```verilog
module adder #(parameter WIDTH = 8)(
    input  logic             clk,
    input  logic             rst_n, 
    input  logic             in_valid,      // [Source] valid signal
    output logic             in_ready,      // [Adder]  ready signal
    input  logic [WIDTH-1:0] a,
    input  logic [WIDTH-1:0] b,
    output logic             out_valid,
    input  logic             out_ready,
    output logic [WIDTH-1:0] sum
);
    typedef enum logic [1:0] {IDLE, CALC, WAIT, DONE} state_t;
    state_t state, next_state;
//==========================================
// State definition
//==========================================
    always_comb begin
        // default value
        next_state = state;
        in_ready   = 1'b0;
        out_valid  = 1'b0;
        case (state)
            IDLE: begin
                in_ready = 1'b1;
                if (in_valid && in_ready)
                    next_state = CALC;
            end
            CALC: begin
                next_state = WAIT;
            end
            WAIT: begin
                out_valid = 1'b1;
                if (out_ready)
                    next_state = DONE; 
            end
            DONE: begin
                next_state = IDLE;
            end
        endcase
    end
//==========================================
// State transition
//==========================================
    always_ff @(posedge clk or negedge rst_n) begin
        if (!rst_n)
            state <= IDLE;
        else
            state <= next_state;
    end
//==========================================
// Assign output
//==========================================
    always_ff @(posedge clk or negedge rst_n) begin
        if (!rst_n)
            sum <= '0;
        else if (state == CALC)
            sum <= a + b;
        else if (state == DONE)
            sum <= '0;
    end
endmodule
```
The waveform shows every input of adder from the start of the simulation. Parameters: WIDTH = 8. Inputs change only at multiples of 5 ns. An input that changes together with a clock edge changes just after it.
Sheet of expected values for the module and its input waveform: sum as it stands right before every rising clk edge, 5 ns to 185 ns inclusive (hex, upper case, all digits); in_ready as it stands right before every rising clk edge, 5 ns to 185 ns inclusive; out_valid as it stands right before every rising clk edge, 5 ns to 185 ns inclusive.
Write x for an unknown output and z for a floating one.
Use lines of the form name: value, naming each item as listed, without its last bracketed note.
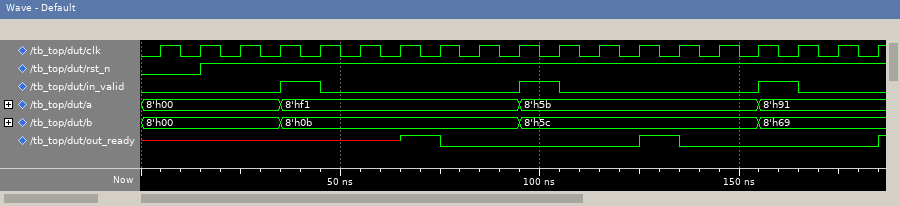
sum as it stands right before every rising clk edge, 5 ns to 185 ns inclusive: 00, 00, 00, 00, 00, 00, FC, FC, FC, 00, 00, 00, B7, B7, B7, 00, 00, 00, FA
in_ready as it stands right before every rising clk edge, 5 ns to 185 ns inclusive: 1 1 1 1 1 0 0 0 0 1 1 0 0 0 0 1 1 0 0
out_valid as it stands right before every rising clk edge, 5 ns to 185 ns inclusive: 0 0 0 0 0 0 1 1 0 0 0 0 1 1 0 0 0 0 1
